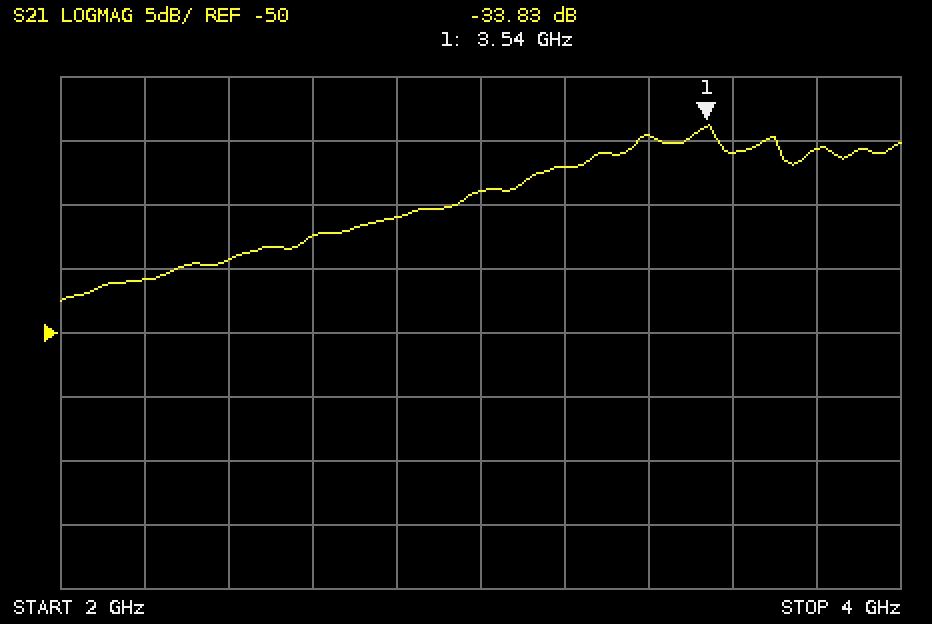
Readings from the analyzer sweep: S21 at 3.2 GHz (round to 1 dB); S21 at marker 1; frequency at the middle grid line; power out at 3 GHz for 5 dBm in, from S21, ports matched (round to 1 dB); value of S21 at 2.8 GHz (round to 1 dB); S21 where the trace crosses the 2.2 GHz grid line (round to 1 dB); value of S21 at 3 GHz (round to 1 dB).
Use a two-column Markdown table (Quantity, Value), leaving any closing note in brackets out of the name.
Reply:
| Quantity | Value |
|---|---|
| S21 at 3.2 GHz | -37 dB |
| S21 at marker 1 | -33.83 dB |
| frequency at the middle grid line | 3 GHz |
| power out at 3 GHz for 5 dBm in, from S21, ports matched | -34 dBm |
| value of S21 at 2.8 GHz | -41 dB |
| S21 where the trace crosses the 2.2 GHz grid line | -46 dB |
| value of S21 at 3 GHz | -39 dB |
